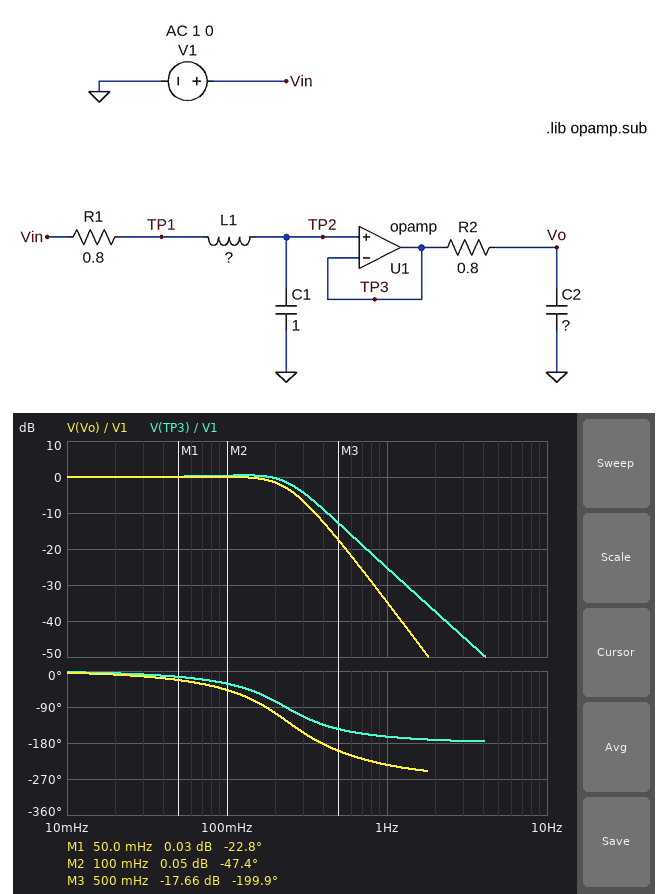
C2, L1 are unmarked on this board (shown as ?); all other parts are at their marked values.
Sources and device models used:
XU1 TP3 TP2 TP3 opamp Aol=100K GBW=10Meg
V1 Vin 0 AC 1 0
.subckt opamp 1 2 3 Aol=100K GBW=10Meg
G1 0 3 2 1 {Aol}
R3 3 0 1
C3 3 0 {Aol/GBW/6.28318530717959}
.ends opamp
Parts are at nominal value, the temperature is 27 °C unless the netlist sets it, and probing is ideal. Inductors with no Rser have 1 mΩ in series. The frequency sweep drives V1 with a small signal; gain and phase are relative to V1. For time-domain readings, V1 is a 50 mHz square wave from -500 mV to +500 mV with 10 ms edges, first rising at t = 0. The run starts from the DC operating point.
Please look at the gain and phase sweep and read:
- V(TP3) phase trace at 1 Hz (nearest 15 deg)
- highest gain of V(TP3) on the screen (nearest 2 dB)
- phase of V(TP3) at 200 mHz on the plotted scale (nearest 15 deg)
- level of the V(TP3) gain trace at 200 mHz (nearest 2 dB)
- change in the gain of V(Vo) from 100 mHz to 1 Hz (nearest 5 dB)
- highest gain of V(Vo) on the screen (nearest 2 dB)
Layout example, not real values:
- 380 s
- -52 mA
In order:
- -165 deg
- 0 dB
- -75 deg
- 0 dB
- -35 dB
- 0 dB
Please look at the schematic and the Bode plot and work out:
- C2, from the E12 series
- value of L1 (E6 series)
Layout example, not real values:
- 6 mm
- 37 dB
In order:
- 560 mF
- 470 mH
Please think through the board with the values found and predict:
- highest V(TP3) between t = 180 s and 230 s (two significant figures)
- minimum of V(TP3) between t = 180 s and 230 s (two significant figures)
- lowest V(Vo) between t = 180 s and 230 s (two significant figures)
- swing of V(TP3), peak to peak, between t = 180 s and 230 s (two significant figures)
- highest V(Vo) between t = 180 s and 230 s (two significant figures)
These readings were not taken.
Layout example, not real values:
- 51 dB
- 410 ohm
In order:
- 600 mV
- -600 mV
- -580 mV
- 1.2 V
- 580 mV
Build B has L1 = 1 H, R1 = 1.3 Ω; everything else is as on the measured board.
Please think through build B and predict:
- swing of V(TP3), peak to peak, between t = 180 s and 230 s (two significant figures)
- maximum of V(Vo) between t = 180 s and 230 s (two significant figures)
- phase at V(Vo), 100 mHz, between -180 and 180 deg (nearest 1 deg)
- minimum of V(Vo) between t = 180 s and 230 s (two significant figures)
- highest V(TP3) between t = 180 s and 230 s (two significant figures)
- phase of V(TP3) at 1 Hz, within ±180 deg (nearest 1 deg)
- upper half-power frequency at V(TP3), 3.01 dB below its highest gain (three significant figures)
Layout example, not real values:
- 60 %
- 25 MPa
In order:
- 1.1 V
- 560 mV
- -69 deg
- -560 mV
- 570 mV
- -168 deg
- 170 mHz
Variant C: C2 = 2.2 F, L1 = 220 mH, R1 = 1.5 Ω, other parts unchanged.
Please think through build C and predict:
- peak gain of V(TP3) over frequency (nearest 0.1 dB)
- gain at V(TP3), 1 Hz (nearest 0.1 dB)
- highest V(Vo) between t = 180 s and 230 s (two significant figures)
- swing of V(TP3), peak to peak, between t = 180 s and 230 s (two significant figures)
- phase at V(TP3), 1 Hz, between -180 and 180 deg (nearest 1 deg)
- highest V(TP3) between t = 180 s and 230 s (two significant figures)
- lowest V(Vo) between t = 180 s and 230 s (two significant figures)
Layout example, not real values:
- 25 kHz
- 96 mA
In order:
- 0 dB
- -21.7 dB
- 490 mV
- 1.0 V
- -129 deg
- 500 mV
- -490 mV
